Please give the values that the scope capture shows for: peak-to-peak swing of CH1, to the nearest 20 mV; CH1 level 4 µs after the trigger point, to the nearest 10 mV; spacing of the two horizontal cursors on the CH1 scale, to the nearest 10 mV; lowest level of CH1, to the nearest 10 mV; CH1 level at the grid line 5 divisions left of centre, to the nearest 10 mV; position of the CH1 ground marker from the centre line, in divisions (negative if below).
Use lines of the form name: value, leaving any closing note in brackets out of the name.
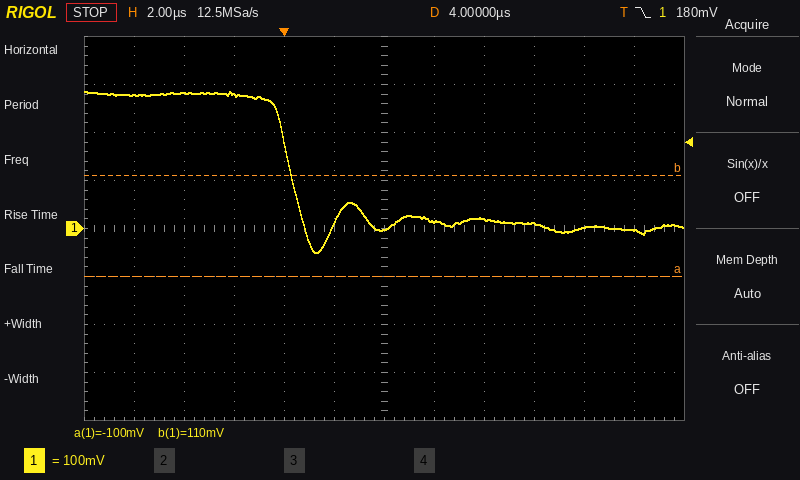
peak-to-peak swing of CH1, to the nearest 20 mV: 340 mV
CH1 level 4 µs after the trigger point, to the nearest 10 mV: 0 mV
spacing of the two horizontal cursors on the CH1 scale, to the nearest 10 mV: 210 mV
lowest level of CH1, to the nearest 10 mV: -50 mV
CH1 level at the grid line 5 divisions left of centre, to the nearest 10 mV: 280 mV
position of the CH1 ground marker from the centre line, in divisions: 0.0 div
